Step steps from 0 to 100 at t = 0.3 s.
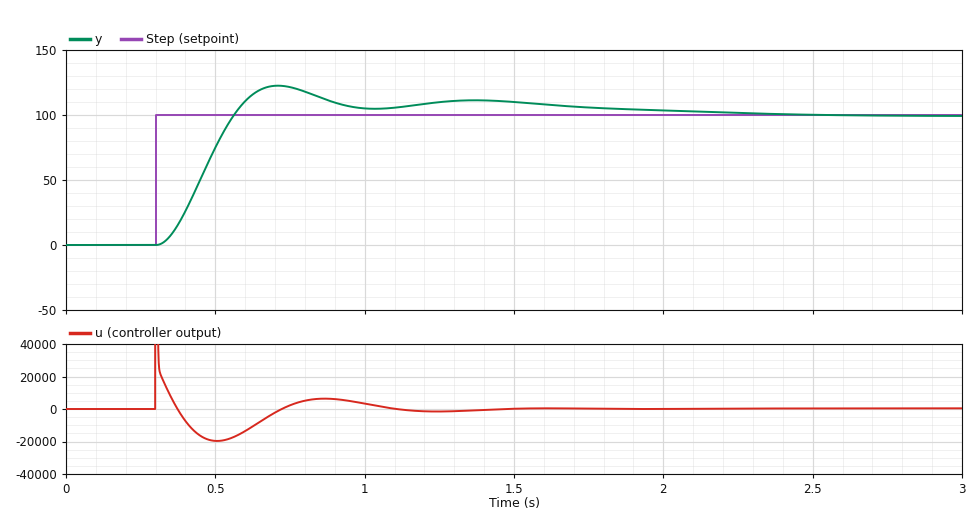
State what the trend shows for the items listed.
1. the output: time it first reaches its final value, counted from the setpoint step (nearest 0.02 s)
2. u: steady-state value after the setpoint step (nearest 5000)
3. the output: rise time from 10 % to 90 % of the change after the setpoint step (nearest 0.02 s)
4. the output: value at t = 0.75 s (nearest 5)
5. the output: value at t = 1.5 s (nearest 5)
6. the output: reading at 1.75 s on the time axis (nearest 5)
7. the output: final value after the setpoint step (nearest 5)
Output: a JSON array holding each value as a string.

["0.26 s", "0", "0.18 s", "120", "110", "105", "100"]
